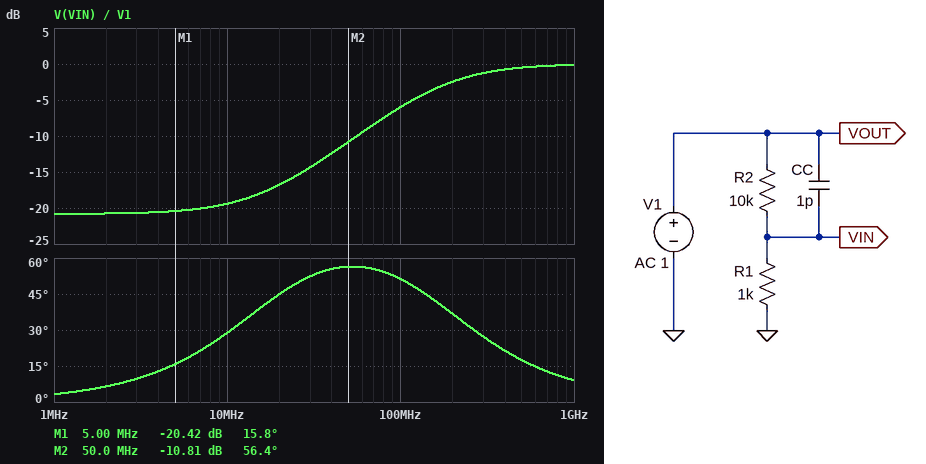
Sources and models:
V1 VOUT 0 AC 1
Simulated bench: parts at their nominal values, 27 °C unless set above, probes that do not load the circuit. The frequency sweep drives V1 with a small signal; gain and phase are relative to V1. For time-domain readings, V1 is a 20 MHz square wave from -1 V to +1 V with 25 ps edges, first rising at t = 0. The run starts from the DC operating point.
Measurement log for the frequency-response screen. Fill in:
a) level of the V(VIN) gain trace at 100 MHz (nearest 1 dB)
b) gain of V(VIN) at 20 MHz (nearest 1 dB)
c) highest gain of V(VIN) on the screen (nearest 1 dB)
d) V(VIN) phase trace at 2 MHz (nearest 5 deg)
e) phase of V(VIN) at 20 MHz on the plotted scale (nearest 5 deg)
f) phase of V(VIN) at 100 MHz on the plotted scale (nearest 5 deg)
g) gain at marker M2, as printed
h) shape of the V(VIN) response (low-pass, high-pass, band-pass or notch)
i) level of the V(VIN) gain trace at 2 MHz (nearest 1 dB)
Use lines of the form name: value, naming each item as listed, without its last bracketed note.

level of the V(VIN) gain trace at 100 MHz: -6 dB
gain of V(VIN) at 20 MHz: -17 dB
highest gain of V(VIN) on the screen: 0 dB
V(VIN) phase trace at 2 MHz: 5 deg
phase of V(VIN) at 20 MHz on the plotted scale: 45 deg
phase of V(VIN) at 100 MHz on the plotted scale: 50 deg
gain at marker M2, as printed: -10.81 dB
shape of the V(VIN) response: high-pass
level of the V(VIN) gain trace at 2 MHz: -21 dB
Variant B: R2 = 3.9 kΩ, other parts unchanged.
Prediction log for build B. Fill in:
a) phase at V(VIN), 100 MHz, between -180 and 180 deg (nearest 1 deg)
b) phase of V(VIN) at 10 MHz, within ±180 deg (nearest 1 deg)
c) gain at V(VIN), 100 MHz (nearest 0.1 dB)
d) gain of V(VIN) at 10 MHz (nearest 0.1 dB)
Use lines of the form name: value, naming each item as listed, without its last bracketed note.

phase at V(VIN), 100 MHz, between -180 and 180 deg: 41 deg
phase of V(VIN) at 10 MHz, within ±180 deg: 11 deg
gain at V(VIN), 100 MHz: -6.3 dB
gain of V(VIN) at 10 MHz: -13.6 dB
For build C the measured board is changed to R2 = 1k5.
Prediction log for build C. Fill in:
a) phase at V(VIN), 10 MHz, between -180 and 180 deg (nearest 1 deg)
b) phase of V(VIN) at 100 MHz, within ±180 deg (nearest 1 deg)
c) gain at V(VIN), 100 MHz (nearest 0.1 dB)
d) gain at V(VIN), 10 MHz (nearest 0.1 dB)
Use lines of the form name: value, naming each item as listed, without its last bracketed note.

phase at V(VIN), 10 MHz, between -180 and 180 deg: 3 deg
phase of V(VIN) at 100 MHz, within ±180 deg: 23 deg
gain at V(VIN), 100 MHz: -5.8 dB
gain at V(VIN), 10 MHz: -7.9 dB
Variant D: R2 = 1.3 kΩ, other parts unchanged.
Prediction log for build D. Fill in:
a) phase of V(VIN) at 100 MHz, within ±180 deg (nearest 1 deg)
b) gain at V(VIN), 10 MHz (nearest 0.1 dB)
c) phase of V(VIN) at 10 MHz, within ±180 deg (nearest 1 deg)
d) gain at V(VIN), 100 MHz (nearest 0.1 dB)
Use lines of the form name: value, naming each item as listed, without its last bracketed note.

phase of V(VIN) at 100 MHz, within ±180 deg: 20 deg
gain at V(VIN), 10 MHz: -7.2 dB
phase of V(VIN) at 10 MHz, within ±180 deg: 3 deg
gain at V(VIN), 100 MHz: -5.5 dB
